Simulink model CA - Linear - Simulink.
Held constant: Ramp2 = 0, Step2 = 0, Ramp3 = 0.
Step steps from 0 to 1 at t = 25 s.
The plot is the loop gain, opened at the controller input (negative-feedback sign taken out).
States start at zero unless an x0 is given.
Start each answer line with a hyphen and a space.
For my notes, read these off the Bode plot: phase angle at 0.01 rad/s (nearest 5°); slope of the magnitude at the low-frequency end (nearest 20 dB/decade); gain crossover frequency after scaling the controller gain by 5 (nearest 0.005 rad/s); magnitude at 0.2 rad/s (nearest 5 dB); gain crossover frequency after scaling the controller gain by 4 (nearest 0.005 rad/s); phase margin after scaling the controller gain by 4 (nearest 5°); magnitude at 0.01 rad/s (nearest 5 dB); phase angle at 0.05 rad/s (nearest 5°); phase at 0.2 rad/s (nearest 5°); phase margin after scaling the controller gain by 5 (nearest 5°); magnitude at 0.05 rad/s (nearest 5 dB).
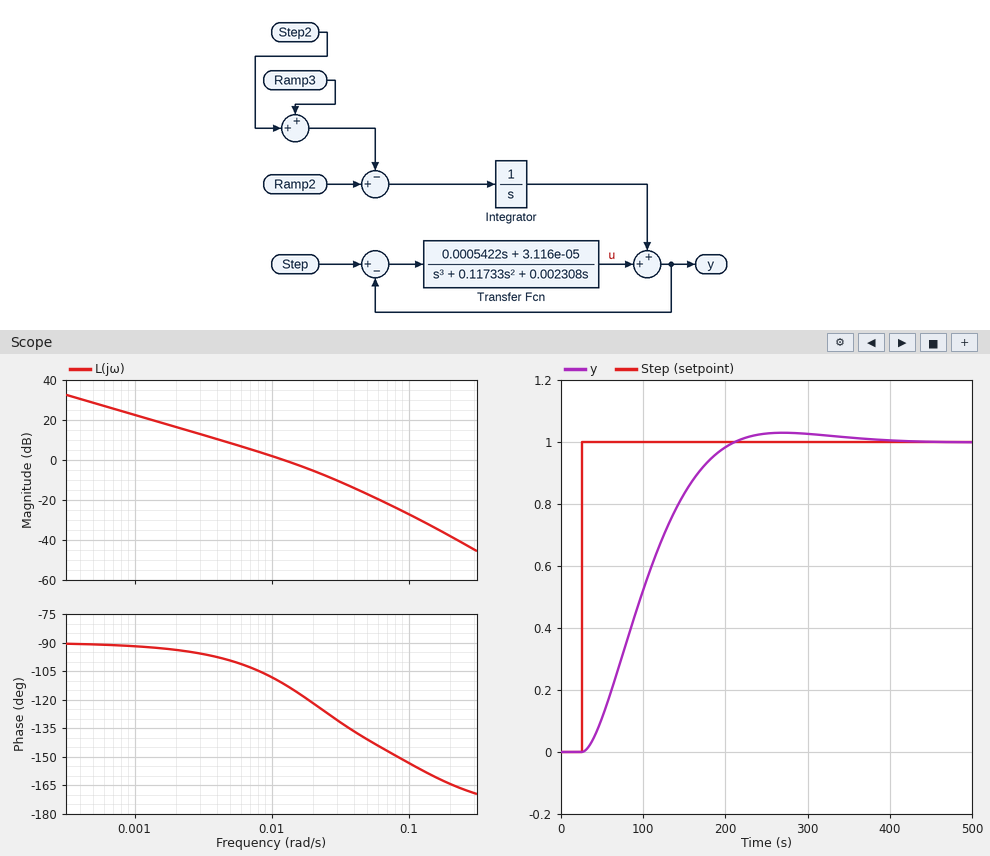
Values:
- -110°
- -20 dB/decade
- 0.040 rad/s
- -40 dB
- 0.035 rad/s
- 45°
- 0 dB
- -140°
- -165°
- 45°
- -15 dB
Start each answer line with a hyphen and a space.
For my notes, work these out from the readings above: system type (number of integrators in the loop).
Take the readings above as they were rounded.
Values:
- 1
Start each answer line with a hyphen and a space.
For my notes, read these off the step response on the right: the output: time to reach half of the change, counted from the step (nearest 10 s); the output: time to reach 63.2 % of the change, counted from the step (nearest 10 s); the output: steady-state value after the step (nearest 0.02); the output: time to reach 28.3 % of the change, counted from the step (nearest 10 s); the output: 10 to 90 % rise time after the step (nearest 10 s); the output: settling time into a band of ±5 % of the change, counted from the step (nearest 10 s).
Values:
- 70 s
- 90 s
- 1.00
- 50 s
- 120 s
- 160 s
